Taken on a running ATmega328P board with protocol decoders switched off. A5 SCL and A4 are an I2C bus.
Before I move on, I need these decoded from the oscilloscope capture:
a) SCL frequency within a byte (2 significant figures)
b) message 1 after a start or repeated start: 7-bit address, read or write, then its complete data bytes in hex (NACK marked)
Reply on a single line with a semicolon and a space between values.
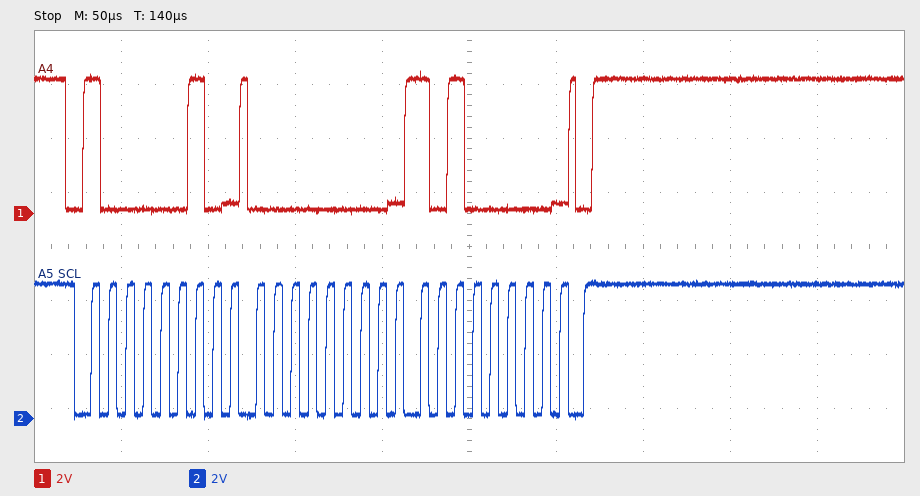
100 kHz; 0x41 write: 00 A0
